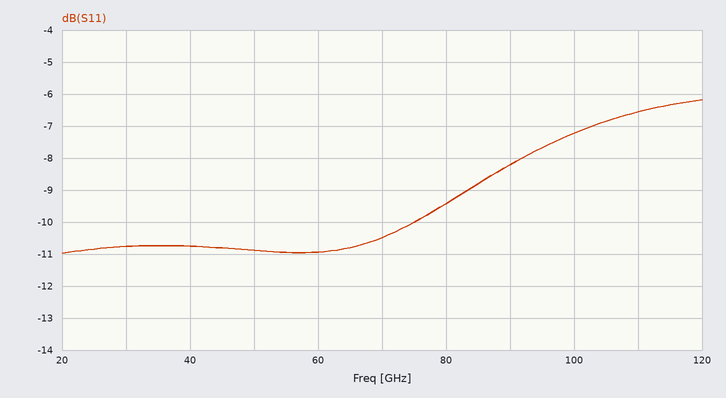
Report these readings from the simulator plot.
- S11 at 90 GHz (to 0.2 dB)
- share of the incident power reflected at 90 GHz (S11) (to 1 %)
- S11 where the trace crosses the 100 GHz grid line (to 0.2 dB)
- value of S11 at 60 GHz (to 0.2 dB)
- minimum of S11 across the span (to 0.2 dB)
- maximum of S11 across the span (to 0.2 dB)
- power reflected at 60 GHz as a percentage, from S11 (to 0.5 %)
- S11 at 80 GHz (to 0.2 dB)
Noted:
-8.2 dB
15 %
-7.2 dB
-11.0 dB
-11.0 dB
-6.2 dB
8.0 %
-9.4 dB
